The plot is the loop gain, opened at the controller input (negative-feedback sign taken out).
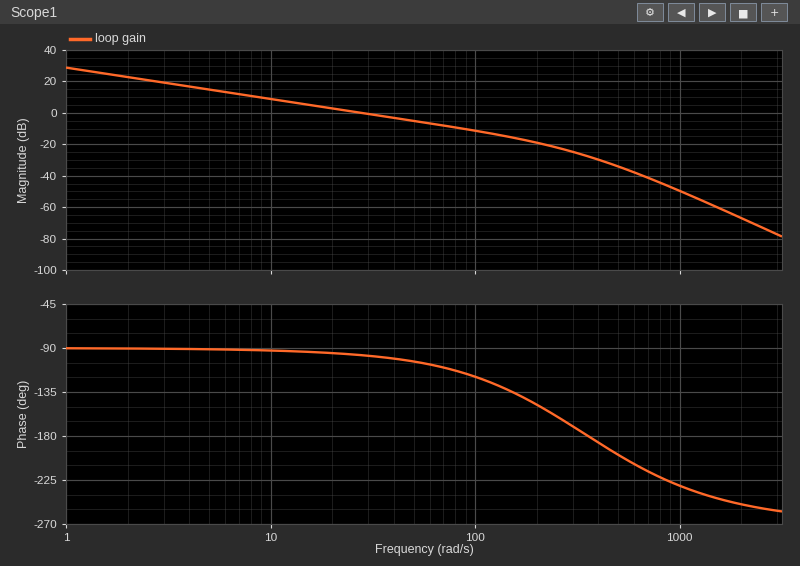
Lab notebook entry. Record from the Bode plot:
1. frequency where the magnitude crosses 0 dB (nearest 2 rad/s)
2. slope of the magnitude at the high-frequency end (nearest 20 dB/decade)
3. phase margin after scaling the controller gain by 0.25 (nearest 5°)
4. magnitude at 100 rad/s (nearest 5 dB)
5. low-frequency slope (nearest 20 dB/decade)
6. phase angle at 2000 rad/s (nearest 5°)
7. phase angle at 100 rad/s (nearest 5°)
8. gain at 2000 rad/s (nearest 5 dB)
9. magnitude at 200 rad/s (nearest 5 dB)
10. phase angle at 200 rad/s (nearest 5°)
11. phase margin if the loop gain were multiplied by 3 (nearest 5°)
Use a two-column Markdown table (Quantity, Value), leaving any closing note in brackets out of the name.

| Quantity | Value |
|---|---|
| frequency where the magnitude crosses 0 dB | 28 rad/s |
| slope of the magnitude at the high-frequency end | -60 dB/decade |
| phase margin after scaling the controller gain by 0.25 | 90° |
| magnitude at 100 rad/s | -10 dB |
| low-frequency slope | -20 dB/decade |
| phase angle at 2000 rad/s | -250° |
| phase angle at 100 rad/s | -120° |
| gain at 2000 rad/s | -65 dB |
| magnitude at 200 rad/s | -20 dB |
| phase angle at 200 rad/s | -150° |
| phase margin if the loop gain were multiplied by 3 | 65° |
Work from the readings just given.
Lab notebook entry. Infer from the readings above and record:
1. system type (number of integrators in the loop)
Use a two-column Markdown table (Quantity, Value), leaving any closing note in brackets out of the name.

| Quantity | Value |
|---|---|
| system type | 1 |
